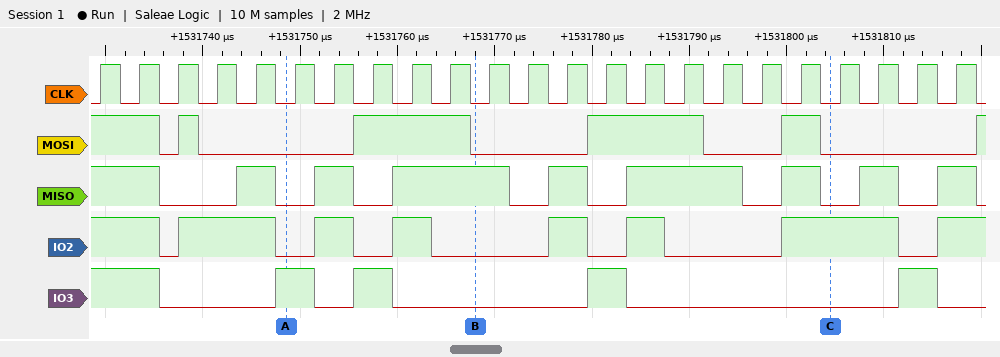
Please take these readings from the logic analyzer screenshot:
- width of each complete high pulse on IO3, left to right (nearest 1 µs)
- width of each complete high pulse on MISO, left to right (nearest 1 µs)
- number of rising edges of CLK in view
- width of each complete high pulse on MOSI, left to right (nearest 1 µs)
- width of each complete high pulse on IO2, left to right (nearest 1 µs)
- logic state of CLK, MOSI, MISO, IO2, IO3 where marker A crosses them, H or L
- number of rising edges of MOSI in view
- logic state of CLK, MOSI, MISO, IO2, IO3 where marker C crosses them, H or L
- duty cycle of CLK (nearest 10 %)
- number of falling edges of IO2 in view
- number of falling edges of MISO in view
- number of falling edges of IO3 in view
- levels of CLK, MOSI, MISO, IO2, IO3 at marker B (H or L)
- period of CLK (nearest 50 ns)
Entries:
4 µs, 4 µs, 4 µs, 4 µs
4 µs, 4 µs, 12 µs, 4 µs, 12 µs, 4 µs, 4 µs, 4 µs
23
2 µs, 12 µs, 12 µs, 4 µs
10 µs, 4 µs, 4 µs, 4 µs, 4 µs, 12 µs
CLK=L, MOSI=L, MISO=L, IO2=L, IO3=H
5
CLK=L, MOSI=L, MISO=L, IO2=H, IO3=L
50 %
7
9
5
CLK=L, MOSI=L, MISO=H, IO2=L, IO3=L
4000 ns
